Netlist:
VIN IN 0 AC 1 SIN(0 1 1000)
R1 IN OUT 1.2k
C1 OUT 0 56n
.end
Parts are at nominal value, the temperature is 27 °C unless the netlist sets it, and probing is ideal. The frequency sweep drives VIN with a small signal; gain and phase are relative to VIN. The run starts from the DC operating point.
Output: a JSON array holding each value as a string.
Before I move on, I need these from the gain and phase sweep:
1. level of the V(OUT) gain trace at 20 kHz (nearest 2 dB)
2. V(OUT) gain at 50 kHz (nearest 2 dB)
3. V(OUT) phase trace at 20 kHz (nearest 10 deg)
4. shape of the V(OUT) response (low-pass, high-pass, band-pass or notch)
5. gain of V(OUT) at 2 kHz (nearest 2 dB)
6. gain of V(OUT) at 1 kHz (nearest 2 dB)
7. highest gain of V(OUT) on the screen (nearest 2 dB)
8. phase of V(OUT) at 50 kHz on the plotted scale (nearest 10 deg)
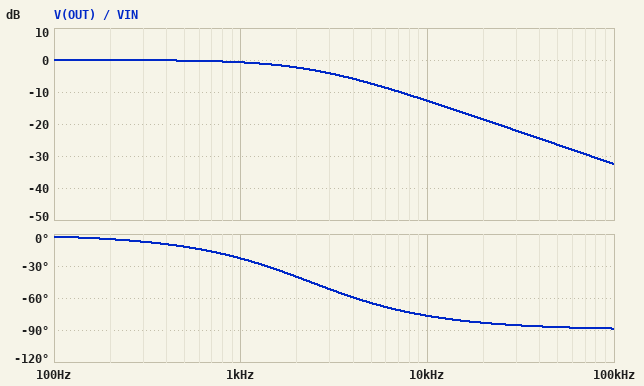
["-18 dB", "-26 dB", "-80 deg", "low-pass", "-2 dB", "0 dB", "0 dB", "-90 deg"]
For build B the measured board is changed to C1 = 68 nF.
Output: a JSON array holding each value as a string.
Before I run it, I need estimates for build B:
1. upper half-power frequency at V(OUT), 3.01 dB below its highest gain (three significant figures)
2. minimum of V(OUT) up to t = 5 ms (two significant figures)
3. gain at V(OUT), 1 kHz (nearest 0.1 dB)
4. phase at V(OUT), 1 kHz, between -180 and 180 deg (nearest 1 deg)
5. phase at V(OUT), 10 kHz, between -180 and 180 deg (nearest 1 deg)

["1.95 kHz", "-890 mV", "-1.0 dB", "-27 deg", "-79 deg"]
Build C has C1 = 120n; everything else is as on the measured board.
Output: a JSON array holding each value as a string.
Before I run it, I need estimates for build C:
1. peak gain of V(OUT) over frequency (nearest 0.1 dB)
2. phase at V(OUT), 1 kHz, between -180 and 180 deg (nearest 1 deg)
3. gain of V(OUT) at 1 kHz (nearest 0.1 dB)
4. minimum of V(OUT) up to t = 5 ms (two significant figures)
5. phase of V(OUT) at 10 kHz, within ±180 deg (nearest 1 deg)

["0 dB", "-42 deg", "-2.6 dB", "-740 mV", "-84 deg"]
